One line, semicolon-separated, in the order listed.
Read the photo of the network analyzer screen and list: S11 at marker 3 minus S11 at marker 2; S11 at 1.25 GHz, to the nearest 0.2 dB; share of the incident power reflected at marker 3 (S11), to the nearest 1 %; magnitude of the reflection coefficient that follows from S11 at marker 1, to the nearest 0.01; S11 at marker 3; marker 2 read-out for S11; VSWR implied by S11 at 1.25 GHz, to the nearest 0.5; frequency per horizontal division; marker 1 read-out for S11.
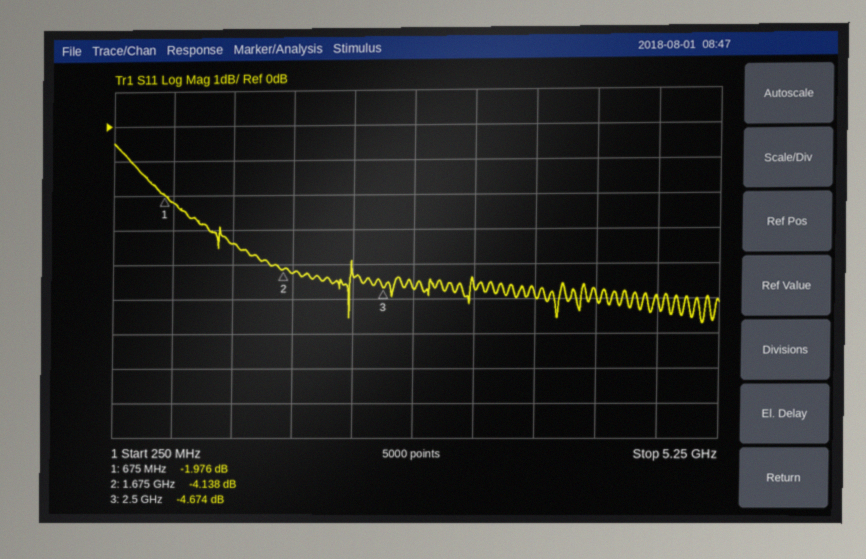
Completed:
-0.536 dB; -3.4 dB; 34 %; 0.80; -4.674 dB; -4.138 dB; 5.0; 500 MHz; -1.976 dB
